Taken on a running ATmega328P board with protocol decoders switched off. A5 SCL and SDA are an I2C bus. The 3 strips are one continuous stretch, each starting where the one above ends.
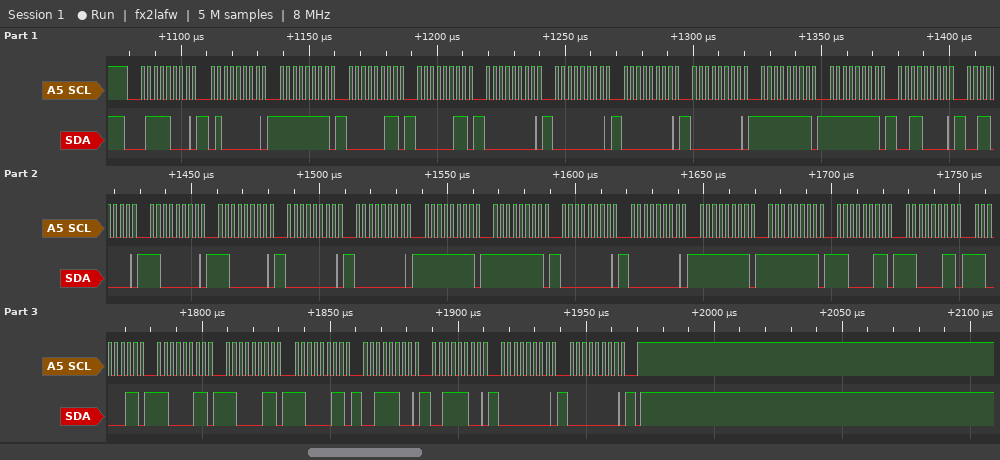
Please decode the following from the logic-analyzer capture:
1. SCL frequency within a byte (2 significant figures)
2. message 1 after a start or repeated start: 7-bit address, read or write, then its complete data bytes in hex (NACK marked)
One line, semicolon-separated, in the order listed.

400 kHz; 0x3C write: 40 FF 03 03 00 00 00 00 FF FF 30 30 C0 C0 00 00 FF FF 00 00 FF FF C3 C3 C3 C3 C3 C3 3C 3C 00 00
